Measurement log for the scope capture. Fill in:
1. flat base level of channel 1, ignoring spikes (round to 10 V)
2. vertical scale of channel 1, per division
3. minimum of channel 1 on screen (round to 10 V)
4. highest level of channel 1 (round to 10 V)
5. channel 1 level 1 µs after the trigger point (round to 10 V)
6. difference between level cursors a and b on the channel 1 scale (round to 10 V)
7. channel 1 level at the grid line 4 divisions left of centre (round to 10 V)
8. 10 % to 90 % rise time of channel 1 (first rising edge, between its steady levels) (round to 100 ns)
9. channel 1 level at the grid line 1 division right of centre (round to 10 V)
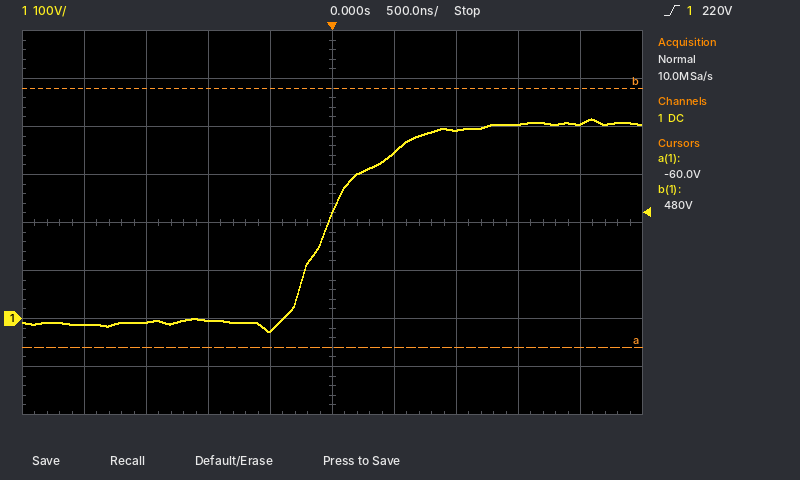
-10 V
100 V
-30 V
420 V
390 V
540 V
-10 V
900 ns
350 V
